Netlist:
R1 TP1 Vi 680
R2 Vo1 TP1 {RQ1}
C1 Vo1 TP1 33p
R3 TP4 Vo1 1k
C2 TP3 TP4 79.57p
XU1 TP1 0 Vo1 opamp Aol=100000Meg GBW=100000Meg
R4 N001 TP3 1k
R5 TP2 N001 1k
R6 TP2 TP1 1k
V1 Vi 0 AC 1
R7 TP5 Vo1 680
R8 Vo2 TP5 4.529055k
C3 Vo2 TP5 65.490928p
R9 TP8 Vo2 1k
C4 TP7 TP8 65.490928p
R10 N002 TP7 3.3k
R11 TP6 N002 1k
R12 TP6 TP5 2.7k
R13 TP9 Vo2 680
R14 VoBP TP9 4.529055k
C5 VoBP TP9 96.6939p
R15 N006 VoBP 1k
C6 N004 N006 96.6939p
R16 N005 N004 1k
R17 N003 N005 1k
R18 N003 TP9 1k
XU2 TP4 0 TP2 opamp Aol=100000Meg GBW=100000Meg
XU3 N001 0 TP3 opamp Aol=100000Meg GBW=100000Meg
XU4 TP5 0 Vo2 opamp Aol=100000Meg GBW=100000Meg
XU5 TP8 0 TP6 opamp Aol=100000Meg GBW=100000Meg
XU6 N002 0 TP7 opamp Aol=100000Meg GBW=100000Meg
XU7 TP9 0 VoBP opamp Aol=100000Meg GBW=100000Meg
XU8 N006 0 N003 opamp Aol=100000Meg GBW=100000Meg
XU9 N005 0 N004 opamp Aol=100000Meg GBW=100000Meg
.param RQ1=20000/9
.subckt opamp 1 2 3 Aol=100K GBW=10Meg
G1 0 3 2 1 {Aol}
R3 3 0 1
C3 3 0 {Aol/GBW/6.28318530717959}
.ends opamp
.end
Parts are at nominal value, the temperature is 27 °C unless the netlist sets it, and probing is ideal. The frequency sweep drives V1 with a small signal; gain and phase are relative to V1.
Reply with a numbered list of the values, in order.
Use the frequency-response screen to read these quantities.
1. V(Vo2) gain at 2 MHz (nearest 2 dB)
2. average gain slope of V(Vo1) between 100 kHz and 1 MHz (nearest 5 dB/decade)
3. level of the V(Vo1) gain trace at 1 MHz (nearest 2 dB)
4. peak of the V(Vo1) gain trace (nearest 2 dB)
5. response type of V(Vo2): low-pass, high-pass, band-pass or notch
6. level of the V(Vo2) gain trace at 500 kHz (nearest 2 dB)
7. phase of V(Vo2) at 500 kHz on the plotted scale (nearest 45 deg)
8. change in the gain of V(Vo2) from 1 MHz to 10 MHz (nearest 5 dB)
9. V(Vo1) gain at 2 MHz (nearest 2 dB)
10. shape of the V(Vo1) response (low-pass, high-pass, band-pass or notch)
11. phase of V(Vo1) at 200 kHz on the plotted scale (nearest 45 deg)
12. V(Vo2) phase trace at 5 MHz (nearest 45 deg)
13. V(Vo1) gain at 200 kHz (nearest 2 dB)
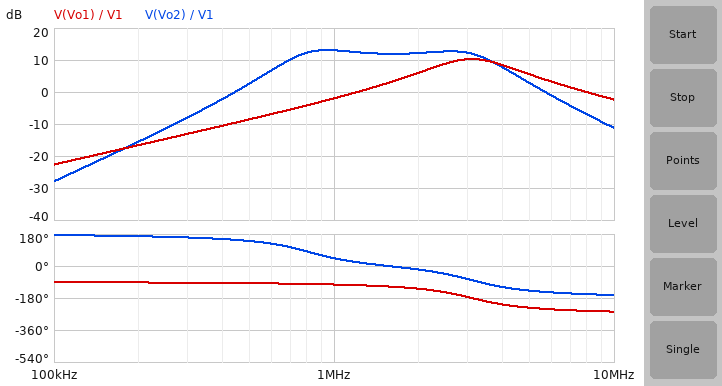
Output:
1. 12 dB
2. 20 dB/decade
3. -2 dB
4. 10 dB
5. band-pass
6. 2 dB
7. 135 deg
8. -25 dB
9. 6 dB
10. band-pass
11. -90 deg
12. -135 deg
13. -16 dB
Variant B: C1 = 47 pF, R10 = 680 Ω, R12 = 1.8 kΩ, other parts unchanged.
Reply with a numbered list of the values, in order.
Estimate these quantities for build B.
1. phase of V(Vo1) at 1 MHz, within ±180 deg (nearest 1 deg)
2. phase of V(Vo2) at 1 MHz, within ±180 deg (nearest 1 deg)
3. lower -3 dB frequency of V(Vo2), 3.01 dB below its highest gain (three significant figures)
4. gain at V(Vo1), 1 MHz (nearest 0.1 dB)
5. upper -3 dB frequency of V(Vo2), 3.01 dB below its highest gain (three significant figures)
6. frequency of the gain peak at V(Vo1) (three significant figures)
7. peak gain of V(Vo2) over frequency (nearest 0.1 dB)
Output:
1. -105 deg
2. 157 deg
3. 2.02 MHz
4. -1.6 dB
5. 2.56 MHz
6. 2.60 MHz
7. 25.6 dB
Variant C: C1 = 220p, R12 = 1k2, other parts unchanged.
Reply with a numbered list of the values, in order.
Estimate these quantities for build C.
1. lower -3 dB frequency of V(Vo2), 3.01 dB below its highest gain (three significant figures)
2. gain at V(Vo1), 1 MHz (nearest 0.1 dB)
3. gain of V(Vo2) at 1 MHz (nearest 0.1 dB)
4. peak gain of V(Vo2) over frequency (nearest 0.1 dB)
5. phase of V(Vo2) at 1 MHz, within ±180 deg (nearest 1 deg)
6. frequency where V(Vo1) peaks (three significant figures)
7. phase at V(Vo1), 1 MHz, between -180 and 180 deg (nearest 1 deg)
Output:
1. 1.09 MHz
2. 5.7 dB
3. 19.5 dB
4. 26.7 dB
5. 96 deg
6. 1.20 MHz
7. -126 deg
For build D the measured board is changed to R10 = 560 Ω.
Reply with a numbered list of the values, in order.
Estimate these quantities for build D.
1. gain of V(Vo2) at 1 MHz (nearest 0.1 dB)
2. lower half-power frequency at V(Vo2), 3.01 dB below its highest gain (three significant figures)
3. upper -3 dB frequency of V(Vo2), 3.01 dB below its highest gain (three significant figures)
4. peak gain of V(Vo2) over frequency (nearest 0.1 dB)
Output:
1. -0.3 dB
2. 1.80 MHz
3. 2.47 MHz
4. 22.5 dB
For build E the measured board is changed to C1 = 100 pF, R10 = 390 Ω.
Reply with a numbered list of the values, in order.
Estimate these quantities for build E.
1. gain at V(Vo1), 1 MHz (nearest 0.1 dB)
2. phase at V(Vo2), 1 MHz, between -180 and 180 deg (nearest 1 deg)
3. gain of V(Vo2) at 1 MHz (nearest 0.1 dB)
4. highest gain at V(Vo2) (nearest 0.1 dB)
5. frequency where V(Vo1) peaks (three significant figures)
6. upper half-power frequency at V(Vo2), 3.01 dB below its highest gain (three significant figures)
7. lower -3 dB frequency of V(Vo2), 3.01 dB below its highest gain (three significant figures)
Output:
1. 0.2 dB
2. 155 deg
3. -2.1 dB
4. 22.3 dB
5. 1.78 MHz
6. 2.53 MHz
7. 1.88 MHz
